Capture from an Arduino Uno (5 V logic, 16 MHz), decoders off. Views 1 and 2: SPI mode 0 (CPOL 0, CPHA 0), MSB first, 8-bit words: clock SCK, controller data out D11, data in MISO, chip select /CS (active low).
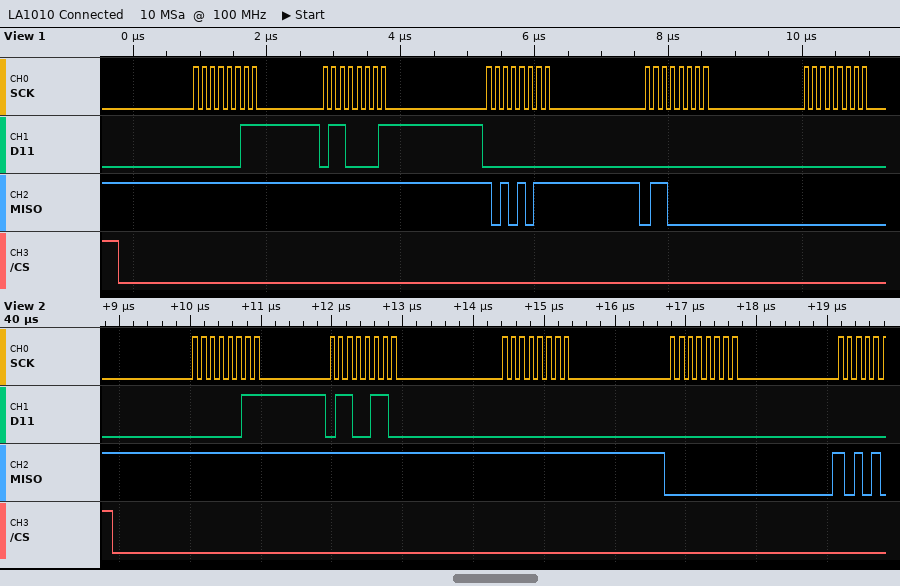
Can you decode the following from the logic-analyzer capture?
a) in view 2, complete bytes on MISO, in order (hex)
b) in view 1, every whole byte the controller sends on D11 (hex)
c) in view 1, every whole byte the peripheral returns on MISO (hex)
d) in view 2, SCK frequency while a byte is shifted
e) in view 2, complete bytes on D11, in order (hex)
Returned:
FF FF FF 00
03 61 00 00 00
FF FF AB 60 00
8 MHz
03 66 00 00
